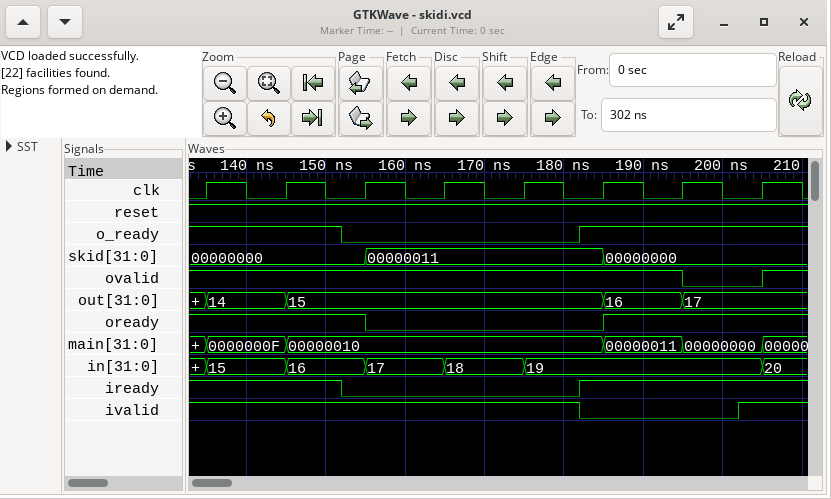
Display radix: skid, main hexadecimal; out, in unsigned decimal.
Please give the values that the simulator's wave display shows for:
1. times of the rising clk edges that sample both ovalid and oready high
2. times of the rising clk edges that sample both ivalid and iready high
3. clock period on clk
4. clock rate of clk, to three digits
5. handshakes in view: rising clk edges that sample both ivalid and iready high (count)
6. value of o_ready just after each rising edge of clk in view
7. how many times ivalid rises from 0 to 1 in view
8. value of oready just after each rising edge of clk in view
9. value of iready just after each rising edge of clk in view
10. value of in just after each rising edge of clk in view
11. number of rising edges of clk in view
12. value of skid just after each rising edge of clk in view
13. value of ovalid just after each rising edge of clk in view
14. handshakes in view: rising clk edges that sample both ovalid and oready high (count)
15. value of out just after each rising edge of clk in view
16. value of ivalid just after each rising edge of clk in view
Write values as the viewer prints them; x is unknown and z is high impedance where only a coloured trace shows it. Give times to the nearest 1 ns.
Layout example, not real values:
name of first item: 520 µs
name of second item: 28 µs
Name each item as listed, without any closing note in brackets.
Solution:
times of the rising clk edges that sample both ovalid and oready high: 135 ns, 145 ns, 155 ns, 195 ns
times of the rising clk edges that sample both ivalid and iready high: 135 ns, 145 ns, 205 ns
clock period on clk: 10 ns
clock rate of clk, to three digits: 100 MHz
handshakes in view: rising clk edges that sample both ivalid and iready high: 3
value of o_ready just after each rising edge of clk in view: 1 1 0 0 0 1 1 1
how many times ivalid rises from 0 to 1 in view: 1
value of oready just after each rising edge of clk in view: 1 1 0 0 0 1 1 1
value of iready just after each rising edge of clk in view: 1 1 0 0 0 1 1 1
value of in just after each rising edge of clk in view: 15, 16, 17, 18, 19, 19, 19, 20
number of rising edges of clk in view: 8
value of skid just after each rising edge of clk in view: 00000000, 00000000, 00000011, 00000011, 00000011, 00000000, 00000000, 00000000
value of ovalid just after each rising edge of clk in view: 1 1 1 1 1 1 0 1
handshakes in view: rising clk edges that sample both ovalid and oready high: 4
value of out just after each rising edge of clk in view: 14, 15, 15, 15, 15, 16, 17, 17
value of ivalid just after each rising edge of clk in view: 1 1 1 1 1 0 0 1
